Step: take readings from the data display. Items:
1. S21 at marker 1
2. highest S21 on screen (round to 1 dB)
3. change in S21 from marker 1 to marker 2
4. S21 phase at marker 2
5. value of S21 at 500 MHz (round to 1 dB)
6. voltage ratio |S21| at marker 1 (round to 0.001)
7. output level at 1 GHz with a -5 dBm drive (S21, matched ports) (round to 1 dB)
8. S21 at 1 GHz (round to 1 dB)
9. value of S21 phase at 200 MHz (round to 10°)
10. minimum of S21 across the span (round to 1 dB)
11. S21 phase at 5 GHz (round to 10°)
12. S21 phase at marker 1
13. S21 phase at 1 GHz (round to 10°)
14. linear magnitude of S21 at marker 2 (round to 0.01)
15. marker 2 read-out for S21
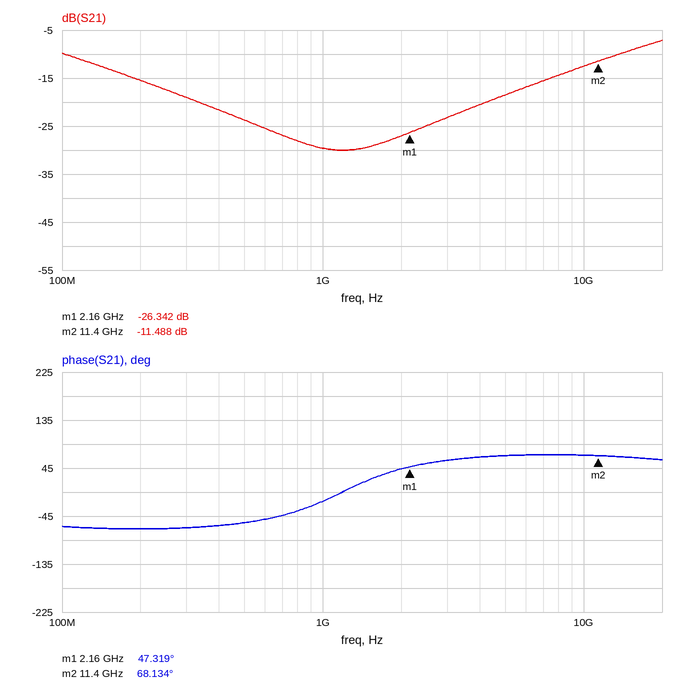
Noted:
-26.342 dB
-7 dB
14.854 dB
68.134°
-24 dB
0.048
-35 dBm
-30 dB
-70°
-30 dB
70°
47.319°
-20°
0.27
-11.488 dB
